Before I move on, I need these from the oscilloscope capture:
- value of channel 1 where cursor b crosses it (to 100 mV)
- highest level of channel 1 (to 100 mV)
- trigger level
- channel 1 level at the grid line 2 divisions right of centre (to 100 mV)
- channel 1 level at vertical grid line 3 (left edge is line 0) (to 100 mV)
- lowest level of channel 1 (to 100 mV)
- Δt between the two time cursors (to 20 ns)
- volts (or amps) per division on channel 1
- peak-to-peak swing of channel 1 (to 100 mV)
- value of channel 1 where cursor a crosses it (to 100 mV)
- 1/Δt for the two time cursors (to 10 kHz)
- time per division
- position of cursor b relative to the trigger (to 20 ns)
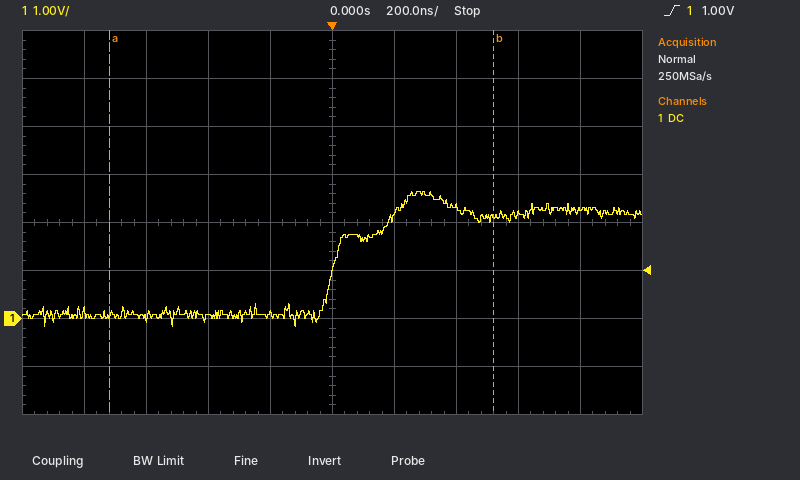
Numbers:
2.1 V
2.6 V
1.00 V
2.3 V
0.0 V
-200 mV
1.24 µs
1 V
2.8 V
100 mV
810 kHz
200 ns
+520 ns
